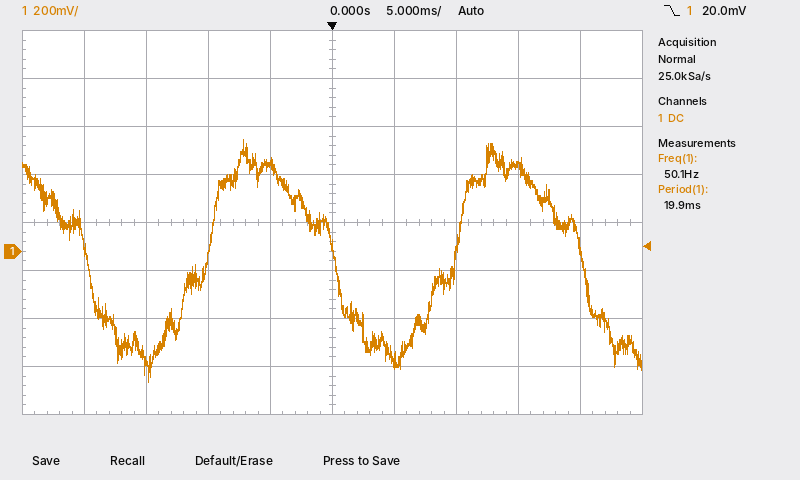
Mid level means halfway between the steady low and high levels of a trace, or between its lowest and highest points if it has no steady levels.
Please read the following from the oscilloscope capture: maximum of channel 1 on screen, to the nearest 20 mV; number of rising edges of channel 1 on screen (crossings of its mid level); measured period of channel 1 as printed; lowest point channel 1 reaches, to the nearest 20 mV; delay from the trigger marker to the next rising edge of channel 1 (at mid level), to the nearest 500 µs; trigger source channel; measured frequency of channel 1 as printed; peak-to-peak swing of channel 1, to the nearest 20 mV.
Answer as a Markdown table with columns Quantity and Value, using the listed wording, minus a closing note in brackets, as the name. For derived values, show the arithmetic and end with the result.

| Quantity | Value |
|---|---|
| maximum of channel 1 on screen, to the nearest 20 mV | 460 mV |
| number of rising edges of channel 1 on screen | 2 |
| measured period of channel 1 as printed | 19.9 ms |
| lowest point channel 1 reaches, to the nearest 20 mV | -540 mV |
| delay from the trigger marker to the next rising edge of channel 1 (at mid level), to the nearest 500 µs | 10.0 ms |
| trigger source channel | channel 1 |
| measured frequency of channel 1 as printed | 50.1 Hz |
| peak-to-peak swing of channel 1, to the nearest 20 mV | 460 mV − (-540 mV) = 1.00 V |
